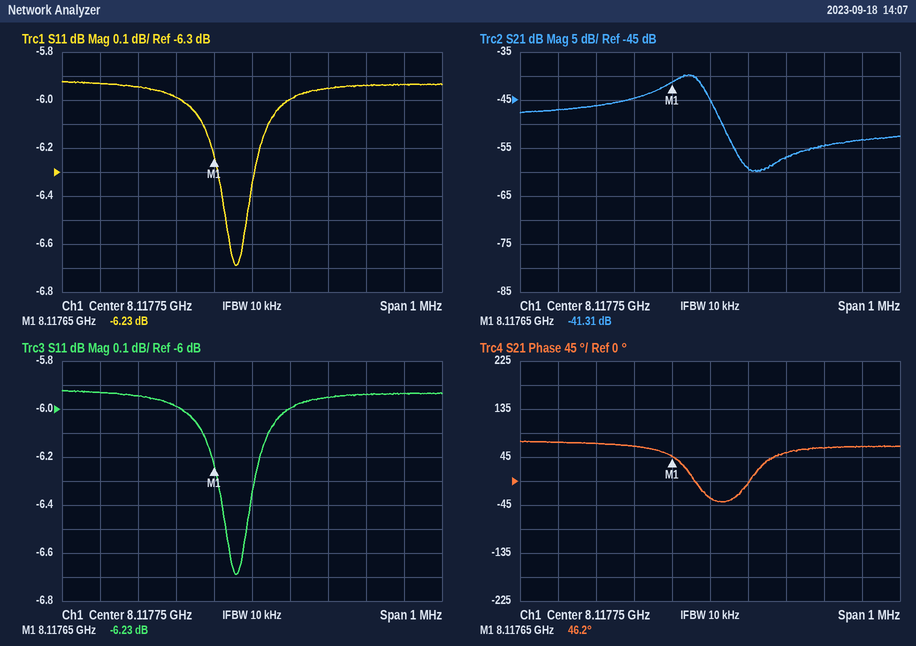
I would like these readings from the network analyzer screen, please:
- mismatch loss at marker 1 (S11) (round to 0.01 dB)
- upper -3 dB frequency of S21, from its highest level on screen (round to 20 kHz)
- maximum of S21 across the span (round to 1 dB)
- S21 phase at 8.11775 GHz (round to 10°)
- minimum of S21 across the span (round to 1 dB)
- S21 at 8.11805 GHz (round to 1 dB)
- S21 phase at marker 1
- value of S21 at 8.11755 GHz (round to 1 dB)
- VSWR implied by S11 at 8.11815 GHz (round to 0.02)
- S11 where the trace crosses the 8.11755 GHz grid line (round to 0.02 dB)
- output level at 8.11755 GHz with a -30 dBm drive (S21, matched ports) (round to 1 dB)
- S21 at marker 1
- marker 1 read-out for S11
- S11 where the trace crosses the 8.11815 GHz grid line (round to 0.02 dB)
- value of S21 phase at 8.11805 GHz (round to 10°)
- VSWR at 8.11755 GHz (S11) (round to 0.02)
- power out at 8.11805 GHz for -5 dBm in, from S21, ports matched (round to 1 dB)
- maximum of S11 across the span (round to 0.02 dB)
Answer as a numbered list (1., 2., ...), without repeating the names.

1. 1.18 dB
2. 8.11774 GHz
3. -40 dB
4. -30°
5. -60 dB
6. -55 dB
7. 46.2°
8. -45 dB
9. 3.04
10. -5.98 dB
11. -75 dBm
12. -41.31 dB
13. -6.23 dB
14. -5.94 dB
15. 60°
16. 3.02
17. -60 dBm
18. -5.92 dB
